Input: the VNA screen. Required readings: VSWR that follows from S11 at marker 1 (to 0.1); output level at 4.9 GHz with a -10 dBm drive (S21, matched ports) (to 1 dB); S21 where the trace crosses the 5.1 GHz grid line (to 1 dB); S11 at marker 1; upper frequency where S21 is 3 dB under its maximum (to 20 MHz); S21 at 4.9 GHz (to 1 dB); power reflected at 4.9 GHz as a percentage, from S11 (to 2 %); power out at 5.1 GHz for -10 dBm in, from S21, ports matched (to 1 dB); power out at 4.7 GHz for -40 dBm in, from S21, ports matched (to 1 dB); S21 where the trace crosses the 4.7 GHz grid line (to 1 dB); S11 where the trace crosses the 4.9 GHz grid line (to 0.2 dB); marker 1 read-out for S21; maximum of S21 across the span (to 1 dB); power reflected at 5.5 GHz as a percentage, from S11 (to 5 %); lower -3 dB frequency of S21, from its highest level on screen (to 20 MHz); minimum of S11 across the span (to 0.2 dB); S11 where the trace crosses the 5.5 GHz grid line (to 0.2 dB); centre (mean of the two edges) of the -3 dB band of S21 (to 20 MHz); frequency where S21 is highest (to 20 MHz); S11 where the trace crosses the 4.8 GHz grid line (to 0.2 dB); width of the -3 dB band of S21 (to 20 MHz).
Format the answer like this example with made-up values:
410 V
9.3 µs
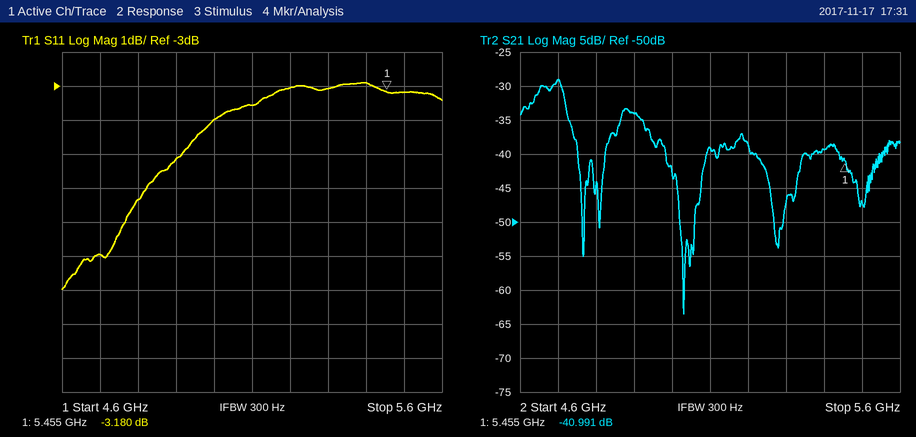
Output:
5.5
-44 dBm
-39 dB
-3.180 dB
4.72 GHz
-34 dB
30 %
-49 dBm
-69 dBm
-29 dB
-5.2 dB
-40.991 dB
-29 dB
50 %
4.64 GHz
-9.0 dB
-3.2 dB
4.68 GHz
4.70 GHz
-6.4 dB
80 MHz
